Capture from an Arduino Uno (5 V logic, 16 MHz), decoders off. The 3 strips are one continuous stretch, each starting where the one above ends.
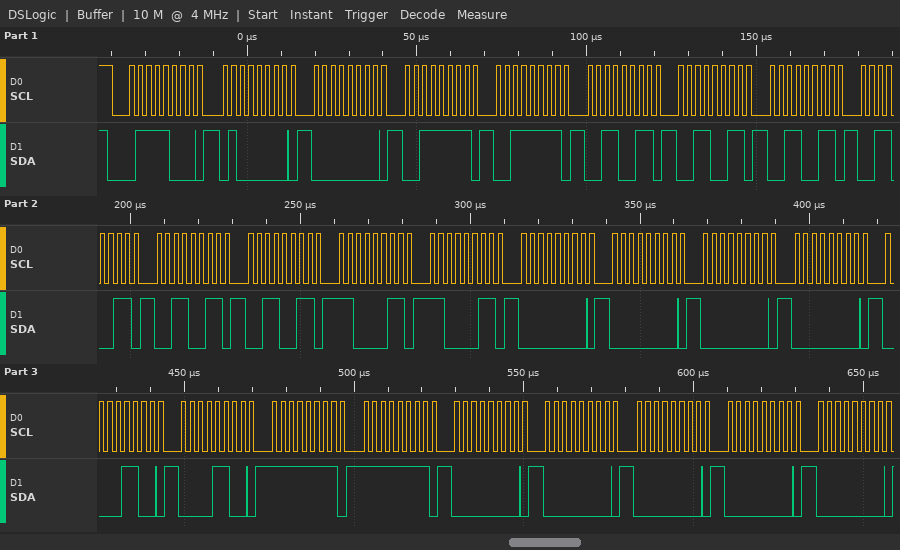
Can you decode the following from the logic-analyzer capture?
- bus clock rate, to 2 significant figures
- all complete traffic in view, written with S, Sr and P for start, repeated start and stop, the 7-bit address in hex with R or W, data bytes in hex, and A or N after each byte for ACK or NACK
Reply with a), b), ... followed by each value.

a) 400 kHz
b) S 3CW A 40 A 00 A 3F A 3F A 33 A 33 A 33 A 33 A 33 A 33 A C3 A C3 A 00 A 00 A 00 A 00 A 0C A 0C A FF A FF A 00 A 00 A 00 A 00 A 00 A
